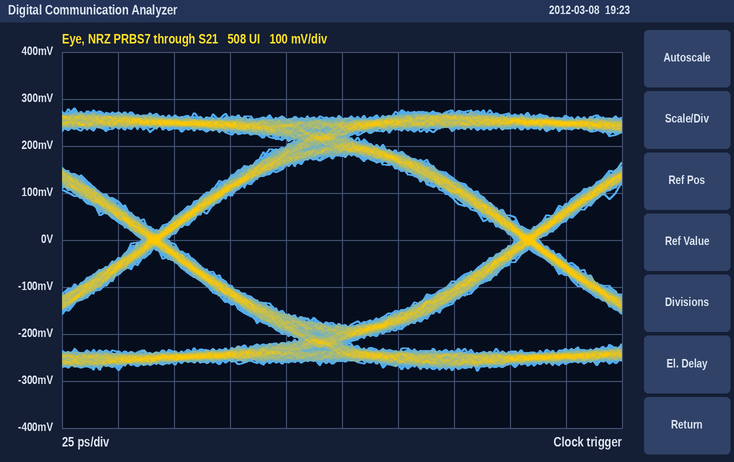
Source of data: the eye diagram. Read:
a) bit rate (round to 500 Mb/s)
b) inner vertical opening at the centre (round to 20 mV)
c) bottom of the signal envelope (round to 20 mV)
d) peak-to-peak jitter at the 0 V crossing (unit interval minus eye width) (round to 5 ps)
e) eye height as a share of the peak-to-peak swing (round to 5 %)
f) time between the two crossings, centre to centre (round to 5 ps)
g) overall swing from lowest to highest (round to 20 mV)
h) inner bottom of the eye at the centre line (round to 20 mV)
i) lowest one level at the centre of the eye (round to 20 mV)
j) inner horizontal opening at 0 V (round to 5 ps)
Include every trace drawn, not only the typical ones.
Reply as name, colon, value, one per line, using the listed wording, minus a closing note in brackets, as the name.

bit rate: 6.0 Gb/s
inner vertical opening at the centre: 360 mV
bottom of the signal envelope: -280 mV
peak-to-peak jitter at the 0 V crossing (unit interval minus eye width): 10 ps
eye height as a share of the peak-to-peak swing: 65 %
time between the two crossings, centre to centre: 165 ps
overall swing from lowest to highest: 560 mV
inner bottom of the eye at the centre line: -180 mV
lowest one level at the centre of the eye: 180 mV
inner horizontal opening at 0 V: 155 ps
